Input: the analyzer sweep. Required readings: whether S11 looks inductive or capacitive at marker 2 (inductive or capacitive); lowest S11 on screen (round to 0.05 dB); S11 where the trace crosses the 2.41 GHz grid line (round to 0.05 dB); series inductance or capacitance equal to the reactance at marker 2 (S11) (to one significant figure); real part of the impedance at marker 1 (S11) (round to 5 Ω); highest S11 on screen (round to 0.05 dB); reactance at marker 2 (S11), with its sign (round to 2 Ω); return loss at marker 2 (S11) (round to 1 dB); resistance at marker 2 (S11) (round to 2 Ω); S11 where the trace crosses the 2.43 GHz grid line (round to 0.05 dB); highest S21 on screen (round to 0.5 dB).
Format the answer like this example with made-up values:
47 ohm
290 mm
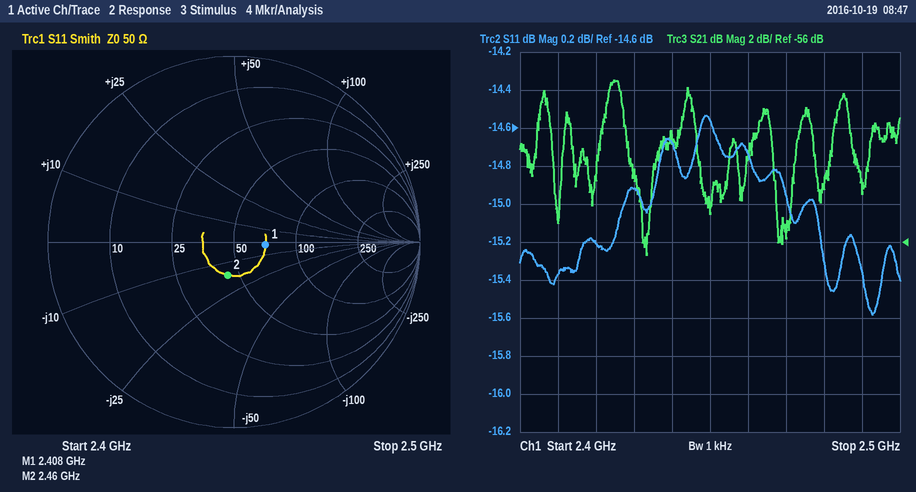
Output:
capacitive
-15.60 dB
-15.35 dB
4 pF
70 Ω
-14.55 dB
-16 Ω
15 dB
44 Ω
-14.90 dB
-47.5 dB
